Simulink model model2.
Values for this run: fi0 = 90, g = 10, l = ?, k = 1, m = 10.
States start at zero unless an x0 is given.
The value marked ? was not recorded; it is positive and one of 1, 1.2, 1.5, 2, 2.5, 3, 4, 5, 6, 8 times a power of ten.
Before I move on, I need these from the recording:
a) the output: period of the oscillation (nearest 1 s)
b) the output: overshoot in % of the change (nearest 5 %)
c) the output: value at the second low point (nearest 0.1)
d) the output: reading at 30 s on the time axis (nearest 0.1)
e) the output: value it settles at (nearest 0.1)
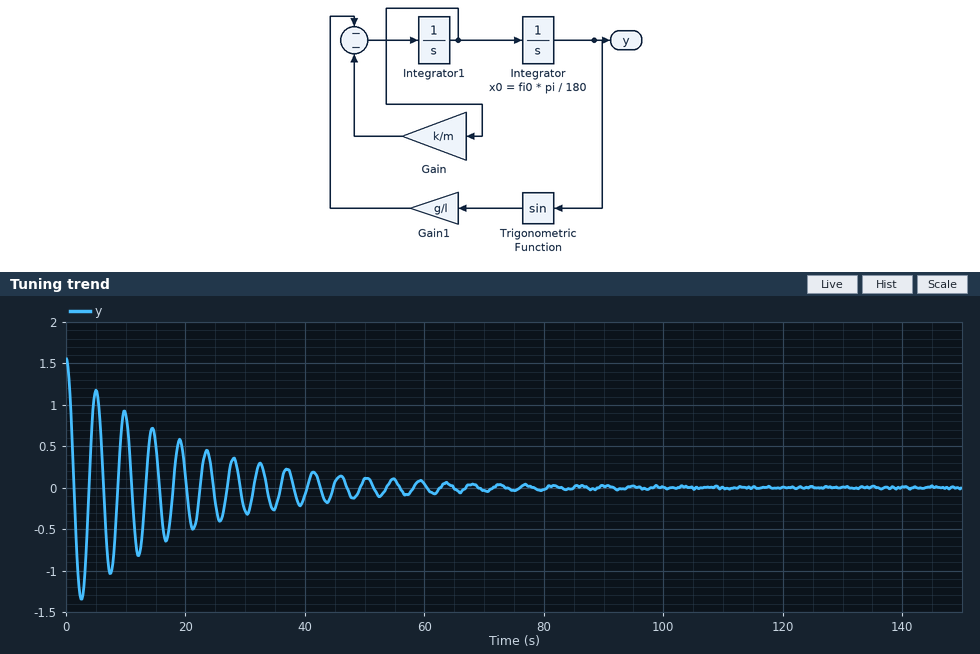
5 s
85 %
-1.0
-0.3
0.0
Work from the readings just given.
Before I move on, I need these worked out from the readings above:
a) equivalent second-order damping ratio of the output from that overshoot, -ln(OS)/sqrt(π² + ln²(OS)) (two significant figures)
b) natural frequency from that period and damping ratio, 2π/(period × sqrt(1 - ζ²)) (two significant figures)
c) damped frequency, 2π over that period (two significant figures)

0.052
1.3 rad/s
1.3 rad/s
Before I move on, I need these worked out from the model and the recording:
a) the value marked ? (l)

5
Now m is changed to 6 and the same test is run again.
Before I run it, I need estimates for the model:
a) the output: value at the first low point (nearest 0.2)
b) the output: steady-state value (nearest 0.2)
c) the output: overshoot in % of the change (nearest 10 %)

-1.2
0.0
80 %
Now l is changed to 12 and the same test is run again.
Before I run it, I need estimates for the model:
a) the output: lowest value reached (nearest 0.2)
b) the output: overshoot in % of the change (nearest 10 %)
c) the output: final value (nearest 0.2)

-1.2
80 %
0.0
